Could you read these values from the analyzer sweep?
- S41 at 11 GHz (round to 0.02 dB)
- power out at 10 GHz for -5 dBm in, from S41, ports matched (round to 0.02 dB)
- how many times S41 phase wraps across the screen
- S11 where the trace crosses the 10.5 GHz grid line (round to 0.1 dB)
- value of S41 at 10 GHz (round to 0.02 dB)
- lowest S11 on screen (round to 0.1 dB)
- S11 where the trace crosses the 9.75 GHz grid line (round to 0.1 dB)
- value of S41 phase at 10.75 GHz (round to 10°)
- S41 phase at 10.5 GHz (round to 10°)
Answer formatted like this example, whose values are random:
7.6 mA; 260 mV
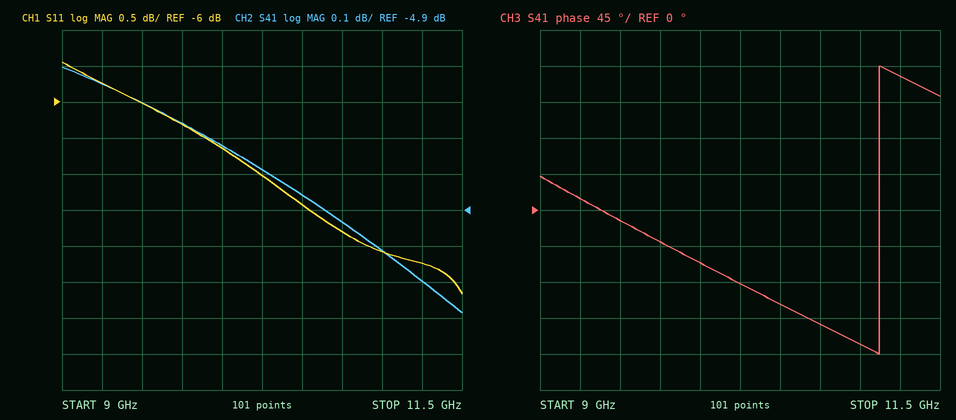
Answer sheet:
-5.02 dB; -9.72 dBm; 1; -7.4 dB; -4.72 dB; -8.7 dB; -6.3 dB; -140°; -120°
